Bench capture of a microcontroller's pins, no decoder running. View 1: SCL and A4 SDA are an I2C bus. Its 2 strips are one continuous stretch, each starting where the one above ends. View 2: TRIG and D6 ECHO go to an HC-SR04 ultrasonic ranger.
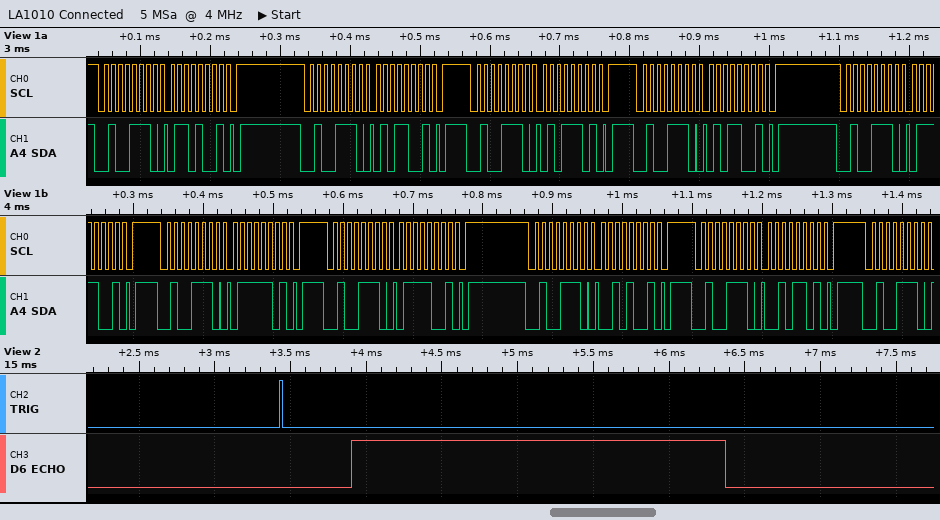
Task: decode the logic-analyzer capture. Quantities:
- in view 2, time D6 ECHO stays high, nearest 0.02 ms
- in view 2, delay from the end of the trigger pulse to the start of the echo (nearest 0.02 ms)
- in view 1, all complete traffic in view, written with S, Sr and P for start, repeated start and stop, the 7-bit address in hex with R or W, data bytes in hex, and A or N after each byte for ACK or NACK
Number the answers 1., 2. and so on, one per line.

1. 2.46 ms
2. 0.46 ms
3. S 27W A 69 A P S 27W A 59 A P S 27W A 5D A P S 27W A 59 A P S 27W A 79 A P S 27W A 7D A P S 27W A 79 A P S 27W A 29 A P S 27W A 2D A P S 27W A
